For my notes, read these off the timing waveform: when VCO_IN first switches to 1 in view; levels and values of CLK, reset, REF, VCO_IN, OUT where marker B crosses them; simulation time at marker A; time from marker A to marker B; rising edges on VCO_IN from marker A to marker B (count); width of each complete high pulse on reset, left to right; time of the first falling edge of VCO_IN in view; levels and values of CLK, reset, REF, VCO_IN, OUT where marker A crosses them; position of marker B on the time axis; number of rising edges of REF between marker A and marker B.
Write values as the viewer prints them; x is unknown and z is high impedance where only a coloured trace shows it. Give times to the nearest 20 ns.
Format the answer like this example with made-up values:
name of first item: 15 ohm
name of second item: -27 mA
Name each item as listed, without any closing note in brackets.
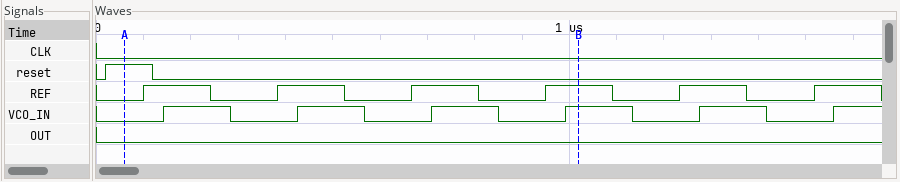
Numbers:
when VCO_IN first switches to 1 in view: 140 ns
levels and values of CLK, reset, REF, VCO_IN, OUT where marker B crosses them: CLK=0, reset=0, REF=1, VCO_IN=1, OUT=0
simulation time at marker A: 60 ns
time from marker A to marker B: 960 ns
rising edges on VCO_IN from marker A to marker B: 4
width of each complete high pulse on reset, left to right: 100 ns
time of the first falling edge of VCO_IN in view: 280 ns
levels and values of CLK, reset, REF, VCO_IN, OUT where marker A crosses them: CLK=0, reset=1, REF=0, VCO_IN=0, OUT=0
position of marker B on the time axis: 1020 ns
number of rising edges of REF between marker A and marker B: 4
